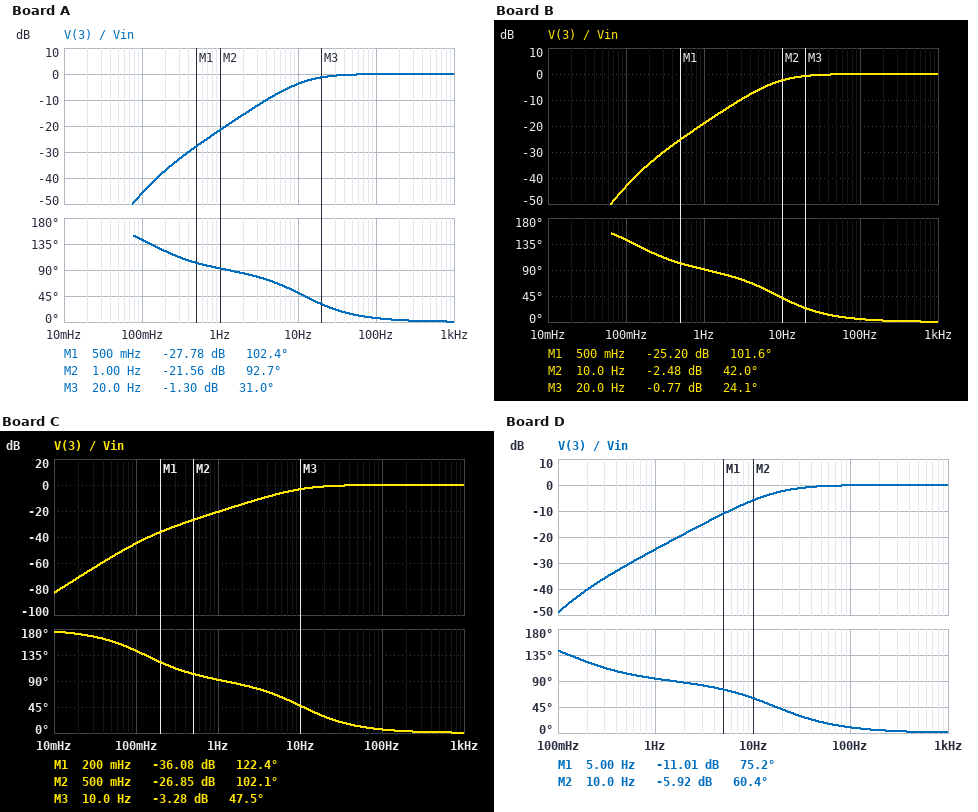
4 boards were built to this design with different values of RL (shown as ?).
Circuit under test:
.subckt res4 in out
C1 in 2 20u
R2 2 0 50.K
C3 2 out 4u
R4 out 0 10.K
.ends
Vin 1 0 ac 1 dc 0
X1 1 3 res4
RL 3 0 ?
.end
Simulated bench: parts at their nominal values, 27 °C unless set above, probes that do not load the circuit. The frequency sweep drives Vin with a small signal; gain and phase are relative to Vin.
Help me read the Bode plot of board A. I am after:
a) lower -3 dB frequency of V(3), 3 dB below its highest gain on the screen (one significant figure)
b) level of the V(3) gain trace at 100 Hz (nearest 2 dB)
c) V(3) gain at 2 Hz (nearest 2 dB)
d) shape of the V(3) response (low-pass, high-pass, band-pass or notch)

10 Hz
0 dB
-16 dB
high-pass
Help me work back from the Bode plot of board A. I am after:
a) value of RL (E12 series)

6.8 kΩ
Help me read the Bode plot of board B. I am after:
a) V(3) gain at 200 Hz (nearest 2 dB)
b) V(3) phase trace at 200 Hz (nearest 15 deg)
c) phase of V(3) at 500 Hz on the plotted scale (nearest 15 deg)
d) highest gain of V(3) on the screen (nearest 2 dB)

0 dB
0 deg
0 deg
0 dB
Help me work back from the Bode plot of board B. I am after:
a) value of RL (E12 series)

12 kΩ
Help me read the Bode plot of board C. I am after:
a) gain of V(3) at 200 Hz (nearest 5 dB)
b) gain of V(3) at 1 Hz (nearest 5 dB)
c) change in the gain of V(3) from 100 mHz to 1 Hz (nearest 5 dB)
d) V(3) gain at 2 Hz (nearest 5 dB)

0 dB
-20 dB
25 dB
-15 dB
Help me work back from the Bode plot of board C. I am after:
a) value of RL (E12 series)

8.2 kΩ
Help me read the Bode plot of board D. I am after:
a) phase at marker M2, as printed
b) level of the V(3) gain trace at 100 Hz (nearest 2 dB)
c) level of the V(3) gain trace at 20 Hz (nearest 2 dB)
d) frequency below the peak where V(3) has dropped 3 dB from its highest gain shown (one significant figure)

60.4 deg
0 dB
-2 dB
20 Hz
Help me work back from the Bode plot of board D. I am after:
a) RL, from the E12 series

3.9 kΩ
